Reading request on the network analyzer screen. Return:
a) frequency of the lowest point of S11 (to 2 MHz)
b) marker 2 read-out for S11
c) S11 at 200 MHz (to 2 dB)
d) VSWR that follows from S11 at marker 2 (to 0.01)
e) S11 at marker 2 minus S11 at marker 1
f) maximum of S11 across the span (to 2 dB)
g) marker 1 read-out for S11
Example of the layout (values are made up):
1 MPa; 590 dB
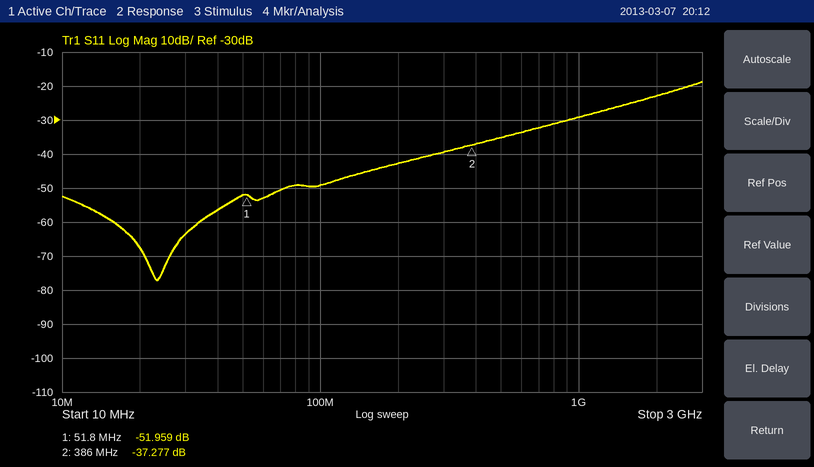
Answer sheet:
24 MHz; -37.277 dB; -42 dB; 1.03; 14.682 dB; -18 dB; -51.959 dB
